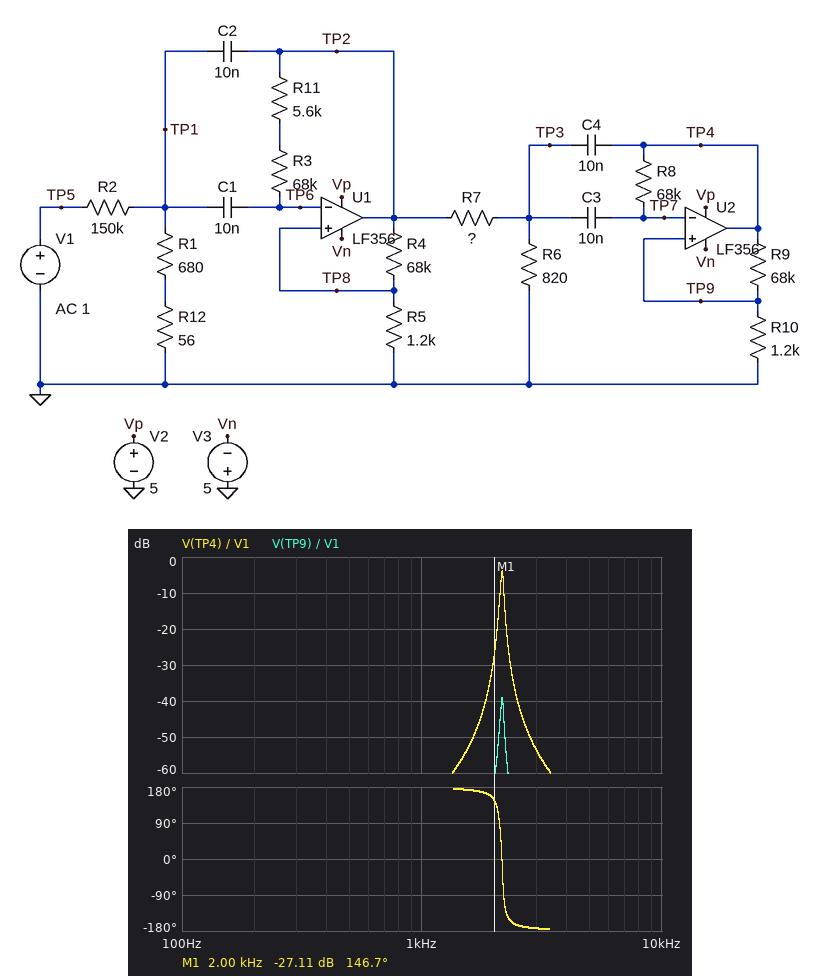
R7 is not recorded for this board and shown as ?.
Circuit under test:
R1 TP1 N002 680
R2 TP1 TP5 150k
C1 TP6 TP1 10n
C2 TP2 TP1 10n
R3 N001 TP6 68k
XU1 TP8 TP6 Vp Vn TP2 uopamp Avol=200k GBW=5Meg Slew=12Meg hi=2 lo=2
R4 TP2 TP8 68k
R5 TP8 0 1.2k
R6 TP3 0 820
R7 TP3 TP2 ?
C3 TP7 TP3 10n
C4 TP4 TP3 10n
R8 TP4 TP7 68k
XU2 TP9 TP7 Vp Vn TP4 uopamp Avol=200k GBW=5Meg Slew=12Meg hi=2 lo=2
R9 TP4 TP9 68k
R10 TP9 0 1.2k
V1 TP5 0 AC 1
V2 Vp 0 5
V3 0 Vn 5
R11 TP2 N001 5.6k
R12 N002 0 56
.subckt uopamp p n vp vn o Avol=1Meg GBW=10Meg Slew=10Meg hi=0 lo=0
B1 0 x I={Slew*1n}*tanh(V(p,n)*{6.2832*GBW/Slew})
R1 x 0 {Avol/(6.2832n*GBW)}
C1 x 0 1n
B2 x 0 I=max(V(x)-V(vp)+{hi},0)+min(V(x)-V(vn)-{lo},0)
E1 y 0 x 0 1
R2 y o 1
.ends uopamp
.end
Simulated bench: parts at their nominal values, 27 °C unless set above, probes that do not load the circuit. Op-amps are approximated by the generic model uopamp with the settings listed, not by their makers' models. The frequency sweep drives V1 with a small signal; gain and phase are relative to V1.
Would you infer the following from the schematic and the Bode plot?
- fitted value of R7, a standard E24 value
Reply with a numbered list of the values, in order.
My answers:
1. 390 kΩ
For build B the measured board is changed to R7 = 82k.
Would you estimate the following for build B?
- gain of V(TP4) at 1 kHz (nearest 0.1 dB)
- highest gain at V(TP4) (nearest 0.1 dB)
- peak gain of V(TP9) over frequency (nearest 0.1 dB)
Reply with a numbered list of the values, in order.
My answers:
1. -55.9 dB
2. 10.4 dB
3. -24.8 dB
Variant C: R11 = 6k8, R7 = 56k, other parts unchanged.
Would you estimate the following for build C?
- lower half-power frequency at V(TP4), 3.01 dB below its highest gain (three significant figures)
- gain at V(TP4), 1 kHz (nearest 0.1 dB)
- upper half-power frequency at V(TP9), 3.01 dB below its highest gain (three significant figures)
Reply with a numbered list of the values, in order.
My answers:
1. 2.13 kHz
2. -52.4 dB
3. 2.16 kHz
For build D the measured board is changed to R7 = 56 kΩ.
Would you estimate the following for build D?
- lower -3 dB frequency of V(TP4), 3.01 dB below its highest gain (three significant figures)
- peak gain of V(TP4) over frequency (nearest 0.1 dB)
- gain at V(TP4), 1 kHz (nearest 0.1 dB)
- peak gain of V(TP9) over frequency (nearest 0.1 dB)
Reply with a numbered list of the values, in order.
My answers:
1. 2.14 kHz
2. 14.0 dB
3. -52.6 dB
4. -21.2 dB
